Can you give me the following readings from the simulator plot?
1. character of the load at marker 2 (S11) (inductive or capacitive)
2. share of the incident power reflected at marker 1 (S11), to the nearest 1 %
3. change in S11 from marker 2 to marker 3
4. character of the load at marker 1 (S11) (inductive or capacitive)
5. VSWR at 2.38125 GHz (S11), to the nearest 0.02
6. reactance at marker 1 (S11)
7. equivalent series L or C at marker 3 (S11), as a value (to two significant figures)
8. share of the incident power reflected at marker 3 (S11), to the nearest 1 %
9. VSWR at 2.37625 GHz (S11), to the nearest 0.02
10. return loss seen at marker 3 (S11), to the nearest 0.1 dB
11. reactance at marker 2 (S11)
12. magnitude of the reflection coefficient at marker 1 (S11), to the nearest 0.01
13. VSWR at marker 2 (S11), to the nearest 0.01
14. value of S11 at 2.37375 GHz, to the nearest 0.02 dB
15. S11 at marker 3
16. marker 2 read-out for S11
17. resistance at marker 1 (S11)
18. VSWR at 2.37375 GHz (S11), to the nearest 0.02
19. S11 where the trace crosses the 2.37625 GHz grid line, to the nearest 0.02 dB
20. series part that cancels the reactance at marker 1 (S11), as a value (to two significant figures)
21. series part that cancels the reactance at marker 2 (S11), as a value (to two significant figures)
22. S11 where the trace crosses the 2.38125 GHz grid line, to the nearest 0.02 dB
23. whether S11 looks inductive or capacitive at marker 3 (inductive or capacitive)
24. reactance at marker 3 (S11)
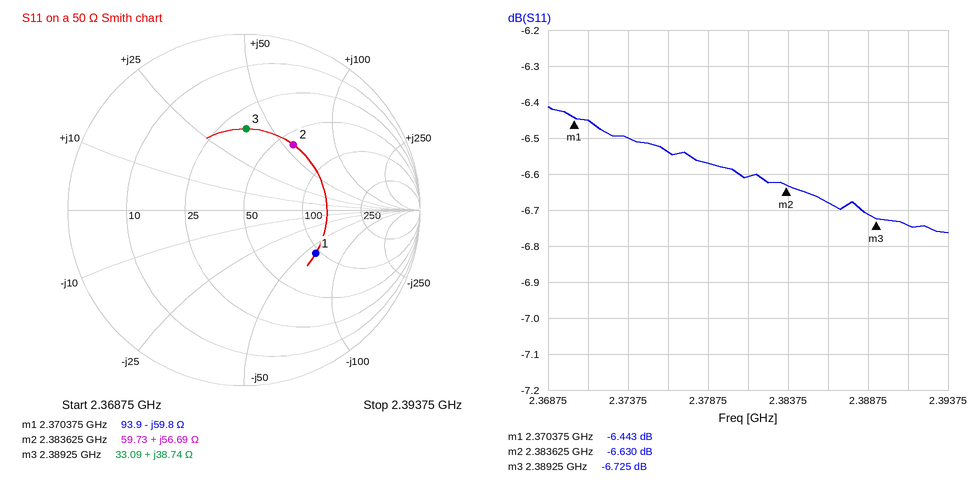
inductive
23 %
-0.095 dB
capacitive
2.76
-59.8 Ω
2.6 nH
21 %
2.78
6.7 dB
+56.69 Ω
0.48
2.75
-6.50 dB
-6.725 dB
-6.630 dB
93.9 Ω
2.80
-6.54 dB
4.0 nH
1.2 pF
-6.60 dB
inductive
+38.74 Ω
